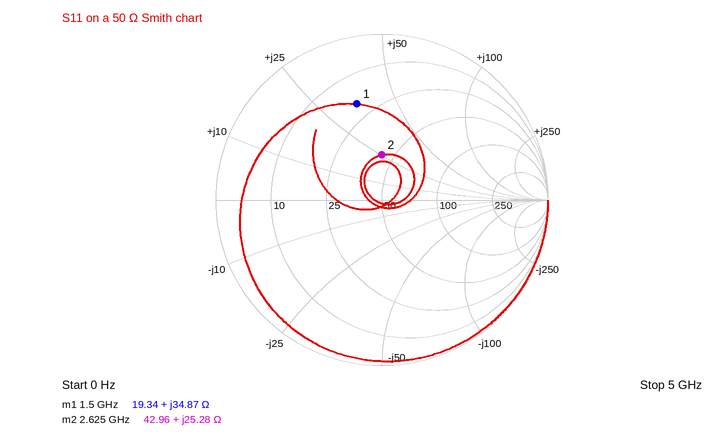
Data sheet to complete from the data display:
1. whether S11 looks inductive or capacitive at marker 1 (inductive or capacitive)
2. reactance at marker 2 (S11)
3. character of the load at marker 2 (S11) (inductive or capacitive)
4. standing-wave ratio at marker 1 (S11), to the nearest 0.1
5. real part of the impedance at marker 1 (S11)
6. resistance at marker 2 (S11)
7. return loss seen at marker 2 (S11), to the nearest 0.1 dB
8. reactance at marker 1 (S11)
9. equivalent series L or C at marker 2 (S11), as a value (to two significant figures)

inductive
+25.28 Ω
inductive
4.0
19.34 Ω
42.96 Ω
11.3 dB
+34.87 Ω
1.5 nH
